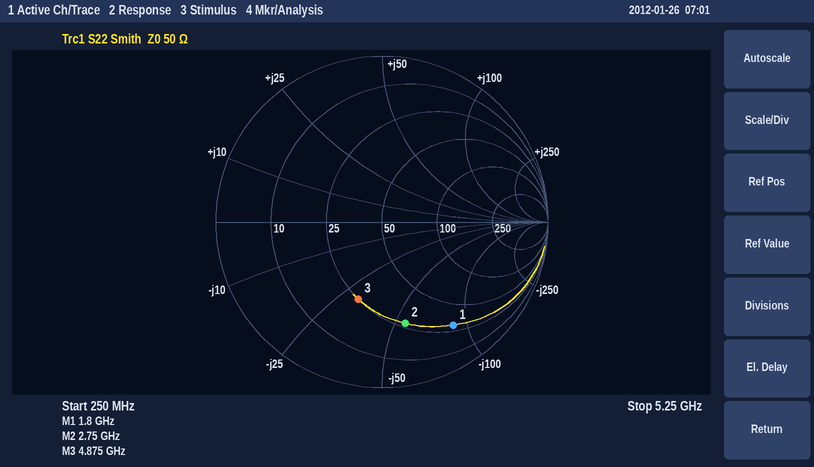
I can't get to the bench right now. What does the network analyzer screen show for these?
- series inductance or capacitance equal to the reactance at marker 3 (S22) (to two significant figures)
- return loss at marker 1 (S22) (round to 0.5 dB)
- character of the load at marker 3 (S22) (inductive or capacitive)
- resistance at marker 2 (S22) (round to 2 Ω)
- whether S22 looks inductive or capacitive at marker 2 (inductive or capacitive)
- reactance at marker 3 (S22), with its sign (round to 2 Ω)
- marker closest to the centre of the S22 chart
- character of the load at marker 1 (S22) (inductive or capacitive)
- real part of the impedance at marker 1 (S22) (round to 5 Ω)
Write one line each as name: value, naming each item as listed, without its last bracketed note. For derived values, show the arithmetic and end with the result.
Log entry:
series inductance or capacitance equal to the reactance at marker 3 (S22): C = 1/(2π × 4.875 GHz × 30 Ω) ≈ 1.1 pF
return loss at marker 1 (S22): 2.5 dB
character of the load at marker 3 (S22): capacitive
resistance at marker 2 (S22): 28 Ω
whether S22 looks inductive or capacitive at marker 2: capacitive
reactance at marker 3 (S22), with its sign: -30 Ω
marker closest to the centre of the S22 chart: marker 3
character of the load at marker 1 (S22): capacitive
real part of the impedance at marker 1 (S22): 30 Ω
